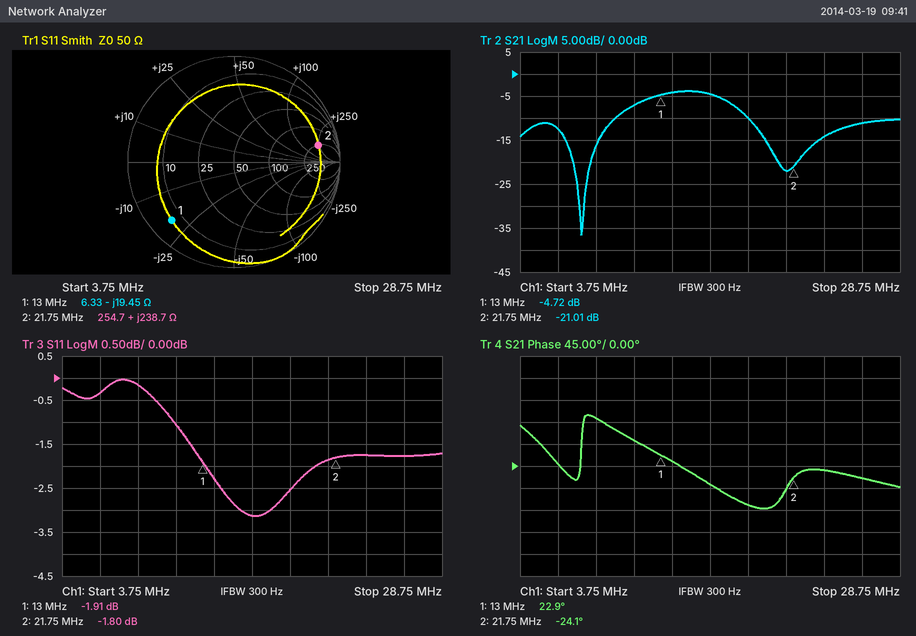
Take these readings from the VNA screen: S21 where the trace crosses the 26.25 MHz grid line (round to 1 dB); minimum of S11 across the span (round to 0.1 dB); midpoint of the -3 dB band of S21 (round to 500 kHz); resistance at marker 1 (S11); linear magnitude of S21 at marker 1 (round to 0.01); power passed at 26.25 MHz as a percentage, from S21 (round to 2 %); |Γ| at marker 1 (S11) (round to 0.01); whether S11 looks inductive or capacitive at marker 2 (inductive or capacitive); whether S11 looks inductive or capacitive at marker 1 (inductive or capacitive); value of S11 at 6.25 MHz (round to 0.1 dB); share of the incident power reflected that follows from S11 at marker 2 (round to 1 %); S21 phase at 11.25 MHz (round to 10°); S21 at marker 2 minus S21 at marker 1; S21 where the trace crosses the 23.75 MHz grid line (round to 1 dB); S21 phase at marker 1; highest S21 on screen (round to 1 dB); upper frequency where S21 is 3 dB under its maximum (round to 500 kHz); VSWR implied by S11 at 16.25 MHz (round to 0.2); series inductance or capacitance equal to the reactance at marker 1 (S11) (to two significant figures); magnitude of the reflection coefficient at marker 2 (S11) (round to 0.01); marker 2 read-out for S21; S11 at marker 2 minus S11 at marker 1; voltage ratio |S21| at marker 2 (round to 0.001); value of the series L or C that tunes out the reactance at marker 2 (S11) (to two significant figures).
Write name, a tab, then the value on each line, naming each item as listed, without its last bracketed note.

S21 where the trace crosses the 26.25 MHz grid line	-11 dB
minimum of S11 across the span	-3.1 dB
midpoint of the -3 dB band of S21	14.5 MHz
resistance at marker 1	6.33 Ω
linear magnitude of S21 at marker 1	0.58
power passed at 26.25 MHz as a percentage, from S21	8 %
|Γ| at marker 1 (S11)	0.80
whether S11 looks inductive or capacitive at marker 2	inductive
whether S11 looks inductive or capacitive at marker 1	capacitive
value of S11 at 6.25 MHz	-0.3 dB
share of the incident power reflected that follows from S11 at marker 2	66 %
S21 phase at 11.25 MHz	50°
S21 at marker 2 minus S21 at marker 1	-16.29 dB
S21 where the trace crosses the 23.75 MHz grid line	-14 dB
S21 phase at marker 1	22.9°
highest S21 on screen	-4 dB
upper frequency where S21 is 3 dB under its maximum	17.5 MHz
VSWR implied by S11 at 16.25 MHz	5.6
series inductance or capacitance equal to the reactance at marker 1 (S11)	630 pF
magnitude of the reflection coefficient at marker 2 (S11)	0.81
marker 2 read-out for S21	-21.01 dB
S11 at marker 2 minus S11 at marker 1	0.11 dB
voltage ratio |S21| at marker 2	0.089
value of the series L or C that tunes out the reactance at marker 2 (S11)	31 pF
